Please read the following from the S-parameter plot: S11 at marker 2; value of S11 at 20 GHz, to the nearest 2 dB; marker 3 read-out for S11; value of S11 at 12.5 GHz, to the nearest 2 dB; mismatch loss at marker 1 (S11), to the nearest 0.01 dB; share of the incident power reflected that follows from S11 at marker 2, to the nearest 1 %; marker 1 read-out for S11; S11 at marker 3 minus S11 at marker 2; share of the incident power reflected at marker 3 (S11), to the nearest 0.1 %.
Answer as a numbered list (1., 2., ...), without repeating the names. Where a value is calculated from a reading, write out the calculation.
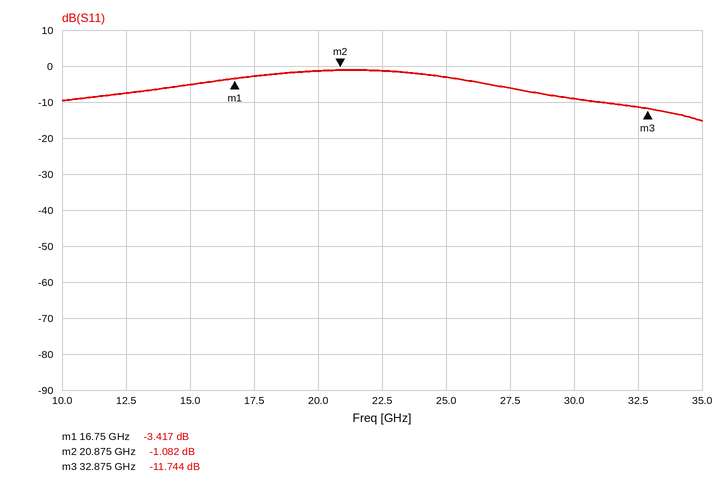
1. -1.082 dB
2. -2 dB
3. -11.744 dB
4. -8 dB
5. −10 log10(1 − 10^(-3.417/10)) ≈ 2.64 dB
6. 10^(-1.082/10) ≈ 78 %
7. -3.417 dB
8. -11.744 − (-1.082) = -10.662 dB
9. 10^(-11.744/10) ≈ 6.7 %
